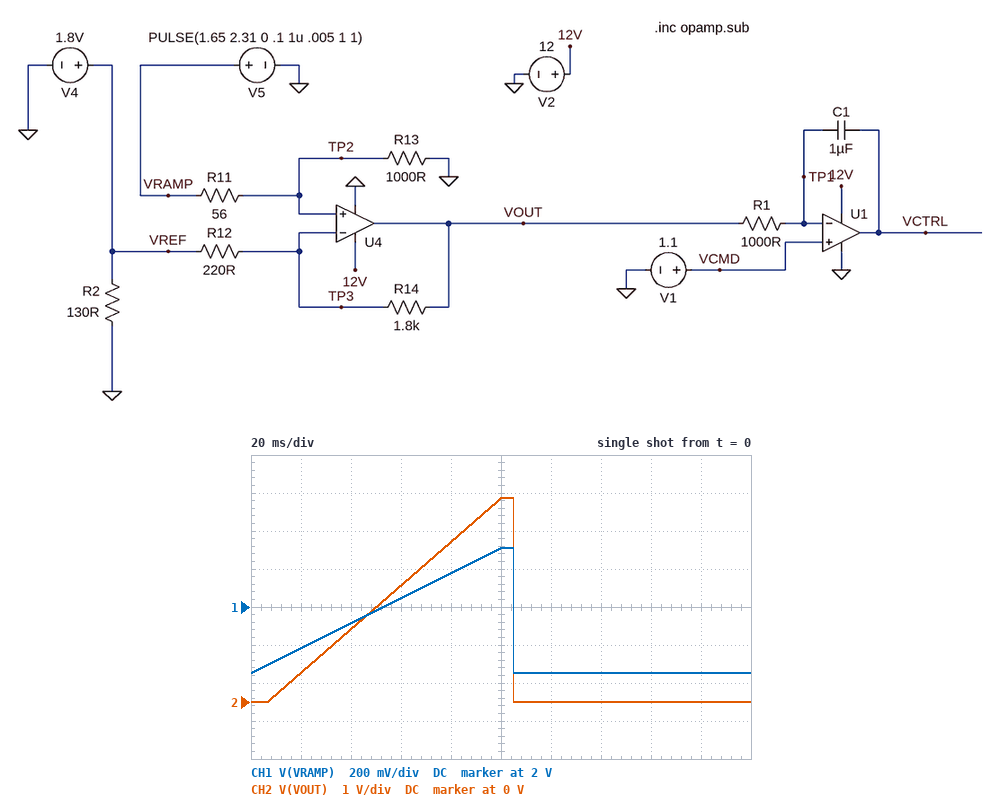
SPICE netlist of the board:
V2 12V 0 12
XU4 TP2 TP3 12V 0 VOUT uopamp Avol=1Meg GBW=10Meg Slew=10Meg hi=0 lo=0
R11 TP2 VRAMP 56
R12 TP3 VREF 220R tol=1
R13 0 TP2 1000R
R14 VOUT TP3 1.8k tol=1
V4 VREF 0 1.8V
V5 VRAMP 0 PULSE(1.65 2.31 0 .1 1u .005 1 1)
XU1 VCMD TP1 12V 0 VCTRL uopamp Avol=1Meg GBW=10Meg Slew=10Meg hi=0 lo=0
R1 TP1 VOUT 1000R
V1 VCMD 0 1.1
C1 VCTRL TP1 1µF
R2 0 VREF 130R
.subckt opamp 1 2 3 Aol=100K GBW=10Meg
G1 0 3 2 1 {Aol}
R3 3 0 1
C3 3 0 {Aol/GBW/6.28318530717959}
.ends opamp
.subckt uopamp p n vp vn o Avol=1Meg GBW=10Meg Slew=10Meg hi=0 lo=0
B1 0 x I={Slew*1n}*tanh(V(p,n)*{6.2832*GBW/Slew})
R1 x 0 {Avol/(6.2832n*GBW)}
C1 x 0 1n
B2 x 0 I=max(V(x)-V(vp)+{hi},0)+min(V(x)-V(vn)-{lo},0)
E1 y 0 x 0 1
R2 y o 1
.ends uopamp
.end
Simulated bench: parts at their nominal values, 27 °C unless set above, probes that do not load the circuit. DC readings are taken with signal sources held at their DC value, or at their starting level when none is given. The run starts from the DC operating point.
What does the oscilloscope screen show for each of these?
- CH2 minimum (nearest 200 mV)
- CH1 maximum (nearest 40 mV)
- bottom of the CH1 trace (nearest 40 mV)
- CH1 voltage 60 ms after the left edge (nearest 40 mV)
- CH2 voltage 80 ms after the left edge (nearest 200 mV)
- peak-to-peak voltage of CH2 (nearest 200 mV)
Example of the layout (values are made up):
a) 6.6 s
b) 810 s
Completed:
a) 0 V
b) 2.32 V
c) 1.64 V
d) 2.04 V
e) 4.2 V
f) 5.4 V
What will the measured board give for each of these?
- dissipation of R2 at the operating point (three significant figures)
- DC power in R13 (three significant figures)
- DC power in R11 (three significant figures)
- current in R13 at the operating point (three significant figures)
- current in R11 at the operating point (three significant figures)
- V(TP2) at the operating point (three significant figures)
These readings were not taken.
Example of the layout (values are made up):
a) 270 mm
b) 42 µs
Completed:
a) 24.9 mW
b) 2.44 mW
c) 137 µW
d) 1.56 mA
e) 1.56 mA
f) 1.56 V
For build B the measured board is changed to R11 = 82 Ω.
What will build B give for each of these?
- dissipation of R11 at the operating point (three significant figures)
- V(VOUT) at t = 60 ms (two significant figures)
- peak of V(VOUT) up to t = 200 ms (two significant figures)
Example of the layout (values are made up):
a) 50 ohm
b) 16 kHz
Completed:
a) 191 µW
b) 2.6 V
c) 4.9 V
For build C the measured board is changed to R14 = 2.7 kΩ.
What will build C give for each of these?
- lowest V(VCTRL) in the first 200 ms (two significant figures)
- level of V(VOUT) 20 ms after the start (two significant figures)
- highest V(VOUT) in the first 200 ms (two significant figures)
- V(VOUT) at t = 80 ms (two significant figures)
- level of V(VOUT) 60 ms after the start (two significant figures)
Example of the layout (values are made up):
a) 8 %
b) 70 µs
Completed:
a) -17 mV
b) 310 mV
c) 6.9 V
d) 5.3 V
e) 3.6 V
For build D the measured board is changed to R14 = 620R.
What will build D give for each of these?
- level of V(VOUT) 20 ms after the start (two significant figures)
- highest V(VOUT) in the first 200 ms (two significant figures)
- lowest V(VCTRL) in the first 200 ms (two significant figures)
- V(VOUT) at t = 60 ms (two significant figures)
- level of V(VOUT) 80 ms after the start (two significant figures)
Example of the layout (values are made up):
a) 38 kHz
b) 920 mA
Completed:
a) 1.4 V
b) 3.3 V
c) -12 mV
d) 2.3 V
e) 2.8 V
